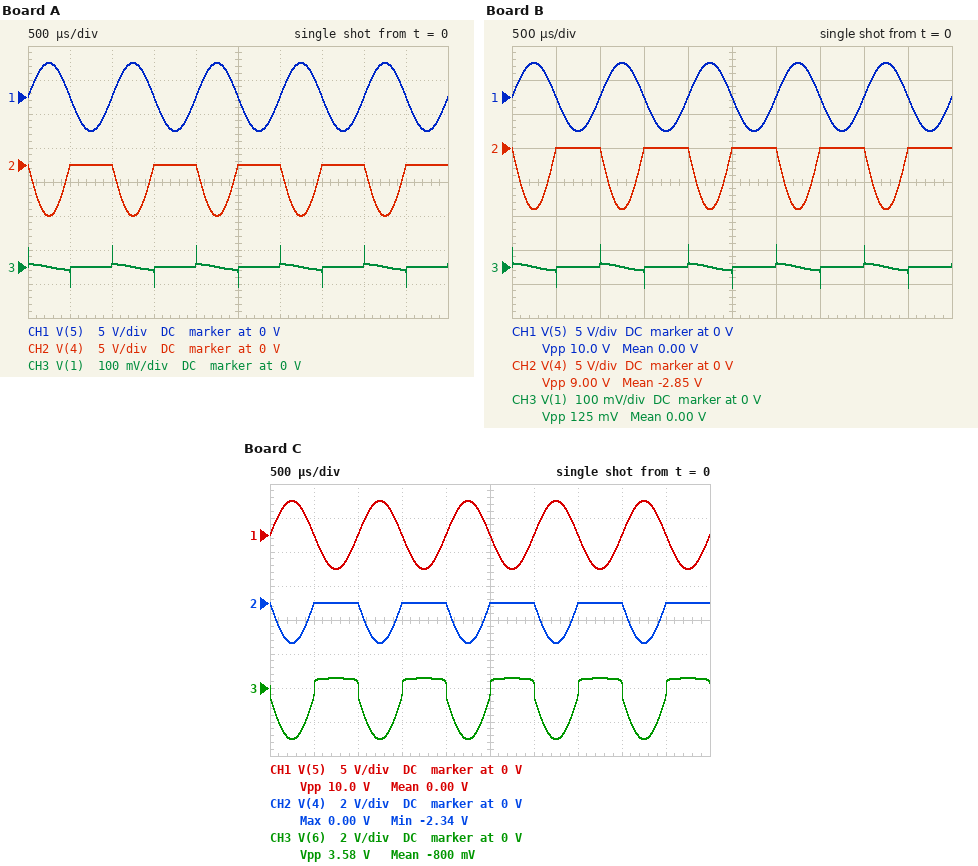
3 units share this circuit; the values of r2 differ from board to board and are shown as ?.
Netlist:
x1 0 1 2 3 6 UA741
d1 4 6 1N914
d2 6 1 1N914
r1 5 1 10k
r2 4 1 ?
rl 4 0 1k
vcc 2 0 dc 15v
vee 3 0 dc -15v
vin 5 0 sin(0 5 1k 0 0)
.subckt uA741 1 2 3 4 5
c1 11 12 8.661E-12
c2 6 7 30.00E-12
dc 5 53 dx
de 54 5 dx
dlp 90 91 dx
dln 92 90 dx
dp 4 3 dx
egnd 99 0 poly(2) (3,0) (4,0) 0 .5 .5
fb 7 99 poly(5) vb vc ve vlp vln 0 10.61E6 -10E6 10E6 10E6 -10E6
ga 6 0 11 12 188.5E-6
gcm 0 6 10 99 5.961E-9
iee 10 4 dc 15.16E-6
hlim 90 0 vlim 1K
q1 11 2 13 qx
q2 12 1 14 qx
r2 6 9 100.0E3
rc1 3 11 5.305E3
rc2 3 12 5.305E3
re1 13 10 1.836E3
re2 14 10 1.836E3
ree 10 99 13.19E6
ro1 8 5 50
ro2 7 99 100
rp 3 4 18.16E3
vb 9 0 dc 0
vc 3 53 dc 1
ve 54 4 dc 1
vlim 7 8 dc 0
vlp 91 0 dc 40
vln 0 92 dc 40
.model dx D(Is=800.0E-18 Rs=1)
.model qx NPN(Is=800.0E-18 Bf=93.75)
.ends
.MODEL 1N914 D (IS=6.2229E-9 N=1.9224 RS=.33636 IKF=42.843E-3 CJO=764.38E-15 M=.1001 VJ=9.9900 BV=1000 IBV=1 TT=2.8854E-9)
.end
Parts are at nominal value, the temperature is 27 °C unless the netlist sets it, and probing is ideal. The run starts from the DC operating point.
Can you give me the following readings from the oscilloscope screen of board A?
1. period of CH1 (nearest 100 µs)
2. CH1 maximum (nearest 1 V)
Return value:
1.0 ms
5 V
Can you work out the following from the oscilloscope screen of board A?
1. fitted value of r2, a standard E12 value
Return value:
15 kΩ
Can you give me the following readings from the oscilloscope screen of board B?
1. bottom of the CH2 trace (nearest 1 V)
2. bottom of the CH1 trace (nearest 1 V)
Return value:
-9 V
-5 V
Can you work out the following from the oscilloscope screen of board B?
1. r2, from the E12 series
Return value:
18 kΩ
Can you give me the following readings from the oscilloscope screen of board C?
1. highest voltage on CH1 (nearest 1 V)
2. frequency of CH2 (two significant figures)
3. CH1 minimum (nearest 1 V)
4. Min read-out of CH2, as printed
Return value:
5 V
1.0 kHz
-5 V
-2.34 V
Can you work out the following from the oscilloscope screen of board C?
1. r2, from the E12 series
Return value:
4.7 kΩ
